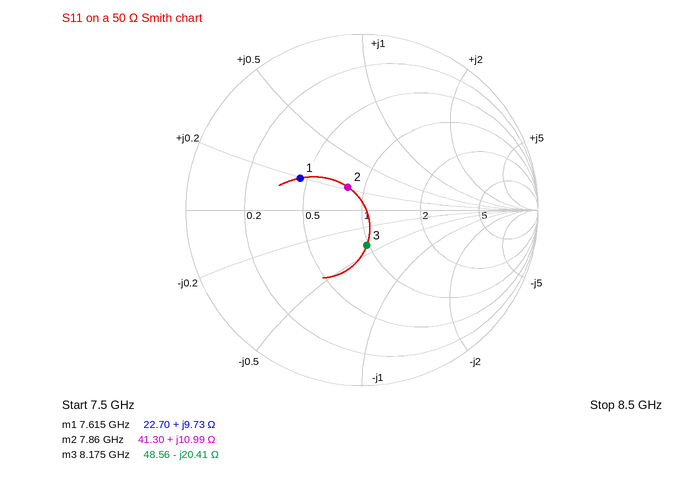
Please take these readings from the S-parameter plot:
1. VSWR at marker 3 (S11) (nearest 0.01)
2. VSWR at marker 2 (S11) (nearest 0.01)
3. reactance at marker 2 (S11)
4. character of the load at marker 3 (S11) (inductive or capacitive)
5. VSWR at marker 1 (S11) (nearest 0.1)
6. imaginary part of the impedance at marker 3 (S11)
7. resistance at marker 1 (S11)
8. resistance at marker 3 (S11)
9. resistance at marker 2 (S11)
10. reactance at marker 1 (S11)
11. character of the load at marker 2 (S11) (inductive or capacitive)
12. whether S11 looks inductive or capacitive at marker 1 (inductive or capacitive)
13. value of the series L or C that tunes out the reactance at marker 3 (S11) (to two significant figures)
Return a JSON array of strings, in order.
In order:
["1.51", "1.36", "+10.99 Ω", "capacitive", "2.3", "-20.41 Ω", "22.70 Ω", "48.56 Ω", "41.30 Ω", "+9.73 Ω", "inductive", "inductive", "400 pH"]
